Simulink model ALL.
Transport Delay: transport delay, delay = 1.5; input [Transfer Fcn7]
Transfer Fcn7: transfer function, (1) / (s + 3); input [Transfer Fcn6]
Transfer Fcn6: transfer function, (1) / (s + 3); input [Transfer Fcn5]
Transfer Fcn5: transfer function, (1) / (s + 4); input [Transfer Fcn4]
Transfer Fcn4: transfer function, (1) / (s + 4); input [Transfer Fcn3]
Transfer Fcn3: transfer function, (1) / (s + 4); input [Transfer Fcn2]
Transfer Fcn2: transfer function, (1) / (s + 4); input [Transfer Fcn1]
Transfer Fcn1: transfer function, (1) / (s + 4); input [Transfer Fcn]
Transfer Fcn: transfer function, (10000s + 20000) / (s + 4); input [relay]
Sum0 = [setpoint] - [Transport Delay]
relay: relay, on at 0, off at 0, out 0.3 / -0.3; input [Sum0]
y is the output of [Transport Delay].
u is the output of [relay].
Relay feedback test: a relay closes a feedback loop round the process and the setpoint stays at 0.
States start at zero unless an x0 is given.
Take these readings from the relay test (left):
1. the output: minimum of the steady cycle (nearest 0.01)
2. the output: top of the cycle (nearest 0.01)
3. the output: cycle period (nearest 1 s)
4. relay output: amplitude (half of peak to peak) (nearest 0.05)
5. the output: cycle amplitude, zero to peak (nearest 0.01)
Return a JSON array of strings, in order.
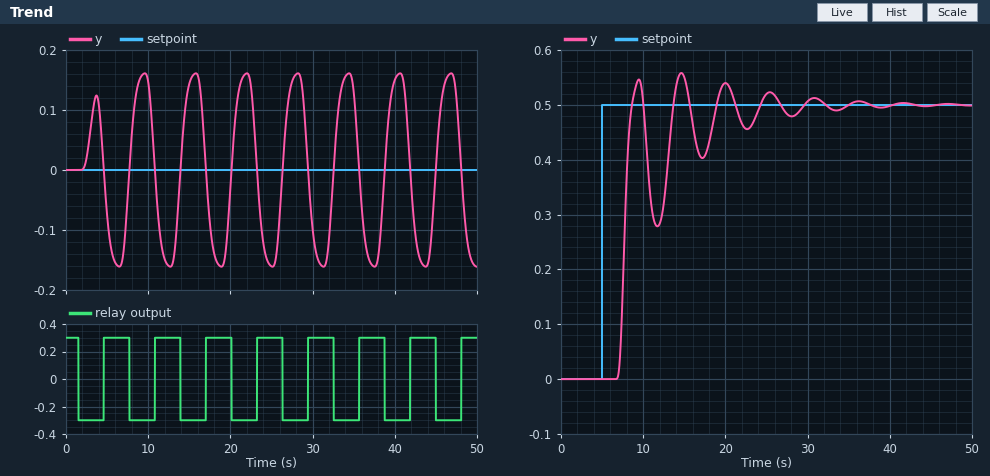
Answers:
["-0.16", "0.16", "6 s", "0.30", "0.16"]
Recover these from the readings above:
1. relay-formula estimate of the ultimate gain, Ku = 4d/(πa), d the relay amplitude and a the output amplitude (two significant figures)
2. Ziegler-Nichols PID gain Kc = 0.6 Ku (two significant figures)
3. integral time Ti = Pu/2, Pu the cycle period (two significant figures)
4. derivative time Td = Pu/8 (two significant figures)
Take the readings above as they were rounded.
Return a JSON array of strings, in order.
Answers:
["2.4", "1.4", "3.0 s", "0.75 s"]
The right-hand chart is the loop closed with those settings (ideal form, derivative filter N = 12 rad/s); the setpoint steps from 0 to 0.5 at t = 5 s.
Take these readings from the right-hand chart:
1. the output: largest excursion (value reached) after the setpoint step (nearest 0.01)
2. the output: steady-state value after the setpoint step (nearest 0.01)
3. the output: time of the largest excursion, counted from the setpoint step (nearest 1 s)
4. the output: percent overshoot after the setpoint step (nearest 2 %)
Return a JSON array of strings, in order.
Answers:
["0.56", "0.50", "10 s", "12 %"]
